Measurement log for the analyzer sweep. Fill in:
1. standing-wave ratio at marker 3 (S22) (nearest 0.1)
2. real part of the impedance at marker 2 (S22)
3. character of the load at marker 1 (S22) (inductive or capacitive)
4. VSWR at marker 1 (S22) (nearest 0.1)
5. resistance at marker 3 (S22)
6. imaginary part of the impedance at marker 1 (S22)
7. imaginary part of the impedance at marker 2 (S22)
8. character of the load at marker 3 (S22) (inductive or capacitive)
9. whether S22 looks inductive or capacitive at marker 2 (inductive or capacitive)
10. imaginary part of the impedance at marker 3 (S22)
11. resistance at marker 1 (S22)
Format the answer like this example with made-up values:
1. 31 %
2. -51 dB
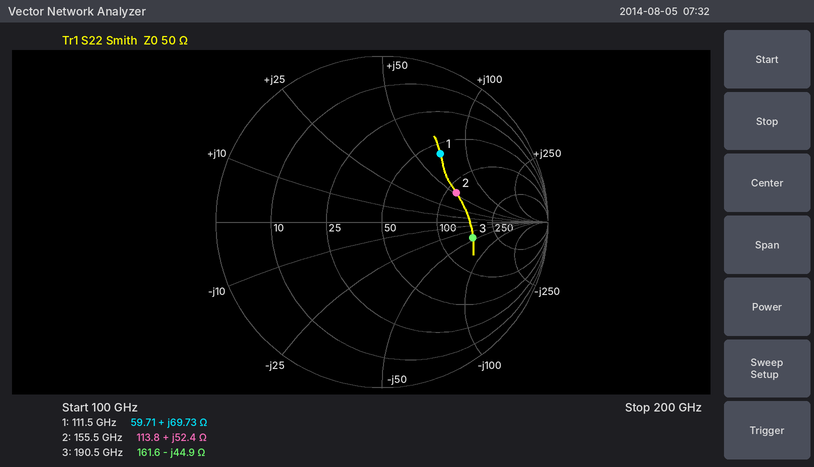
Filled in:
1. 3.5
2. 113.8 Ω
3. inductive
4. 3.4
5. 161.6 Ω
6. +69.73 Ω
7. +52.4 Ω
8. capacitive
9. inductive
10. -44.9 Ω
11. 59.71 Ω
